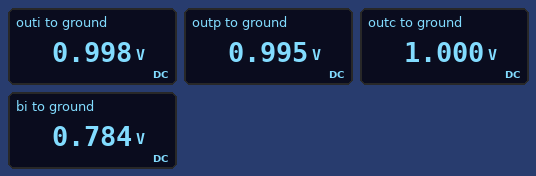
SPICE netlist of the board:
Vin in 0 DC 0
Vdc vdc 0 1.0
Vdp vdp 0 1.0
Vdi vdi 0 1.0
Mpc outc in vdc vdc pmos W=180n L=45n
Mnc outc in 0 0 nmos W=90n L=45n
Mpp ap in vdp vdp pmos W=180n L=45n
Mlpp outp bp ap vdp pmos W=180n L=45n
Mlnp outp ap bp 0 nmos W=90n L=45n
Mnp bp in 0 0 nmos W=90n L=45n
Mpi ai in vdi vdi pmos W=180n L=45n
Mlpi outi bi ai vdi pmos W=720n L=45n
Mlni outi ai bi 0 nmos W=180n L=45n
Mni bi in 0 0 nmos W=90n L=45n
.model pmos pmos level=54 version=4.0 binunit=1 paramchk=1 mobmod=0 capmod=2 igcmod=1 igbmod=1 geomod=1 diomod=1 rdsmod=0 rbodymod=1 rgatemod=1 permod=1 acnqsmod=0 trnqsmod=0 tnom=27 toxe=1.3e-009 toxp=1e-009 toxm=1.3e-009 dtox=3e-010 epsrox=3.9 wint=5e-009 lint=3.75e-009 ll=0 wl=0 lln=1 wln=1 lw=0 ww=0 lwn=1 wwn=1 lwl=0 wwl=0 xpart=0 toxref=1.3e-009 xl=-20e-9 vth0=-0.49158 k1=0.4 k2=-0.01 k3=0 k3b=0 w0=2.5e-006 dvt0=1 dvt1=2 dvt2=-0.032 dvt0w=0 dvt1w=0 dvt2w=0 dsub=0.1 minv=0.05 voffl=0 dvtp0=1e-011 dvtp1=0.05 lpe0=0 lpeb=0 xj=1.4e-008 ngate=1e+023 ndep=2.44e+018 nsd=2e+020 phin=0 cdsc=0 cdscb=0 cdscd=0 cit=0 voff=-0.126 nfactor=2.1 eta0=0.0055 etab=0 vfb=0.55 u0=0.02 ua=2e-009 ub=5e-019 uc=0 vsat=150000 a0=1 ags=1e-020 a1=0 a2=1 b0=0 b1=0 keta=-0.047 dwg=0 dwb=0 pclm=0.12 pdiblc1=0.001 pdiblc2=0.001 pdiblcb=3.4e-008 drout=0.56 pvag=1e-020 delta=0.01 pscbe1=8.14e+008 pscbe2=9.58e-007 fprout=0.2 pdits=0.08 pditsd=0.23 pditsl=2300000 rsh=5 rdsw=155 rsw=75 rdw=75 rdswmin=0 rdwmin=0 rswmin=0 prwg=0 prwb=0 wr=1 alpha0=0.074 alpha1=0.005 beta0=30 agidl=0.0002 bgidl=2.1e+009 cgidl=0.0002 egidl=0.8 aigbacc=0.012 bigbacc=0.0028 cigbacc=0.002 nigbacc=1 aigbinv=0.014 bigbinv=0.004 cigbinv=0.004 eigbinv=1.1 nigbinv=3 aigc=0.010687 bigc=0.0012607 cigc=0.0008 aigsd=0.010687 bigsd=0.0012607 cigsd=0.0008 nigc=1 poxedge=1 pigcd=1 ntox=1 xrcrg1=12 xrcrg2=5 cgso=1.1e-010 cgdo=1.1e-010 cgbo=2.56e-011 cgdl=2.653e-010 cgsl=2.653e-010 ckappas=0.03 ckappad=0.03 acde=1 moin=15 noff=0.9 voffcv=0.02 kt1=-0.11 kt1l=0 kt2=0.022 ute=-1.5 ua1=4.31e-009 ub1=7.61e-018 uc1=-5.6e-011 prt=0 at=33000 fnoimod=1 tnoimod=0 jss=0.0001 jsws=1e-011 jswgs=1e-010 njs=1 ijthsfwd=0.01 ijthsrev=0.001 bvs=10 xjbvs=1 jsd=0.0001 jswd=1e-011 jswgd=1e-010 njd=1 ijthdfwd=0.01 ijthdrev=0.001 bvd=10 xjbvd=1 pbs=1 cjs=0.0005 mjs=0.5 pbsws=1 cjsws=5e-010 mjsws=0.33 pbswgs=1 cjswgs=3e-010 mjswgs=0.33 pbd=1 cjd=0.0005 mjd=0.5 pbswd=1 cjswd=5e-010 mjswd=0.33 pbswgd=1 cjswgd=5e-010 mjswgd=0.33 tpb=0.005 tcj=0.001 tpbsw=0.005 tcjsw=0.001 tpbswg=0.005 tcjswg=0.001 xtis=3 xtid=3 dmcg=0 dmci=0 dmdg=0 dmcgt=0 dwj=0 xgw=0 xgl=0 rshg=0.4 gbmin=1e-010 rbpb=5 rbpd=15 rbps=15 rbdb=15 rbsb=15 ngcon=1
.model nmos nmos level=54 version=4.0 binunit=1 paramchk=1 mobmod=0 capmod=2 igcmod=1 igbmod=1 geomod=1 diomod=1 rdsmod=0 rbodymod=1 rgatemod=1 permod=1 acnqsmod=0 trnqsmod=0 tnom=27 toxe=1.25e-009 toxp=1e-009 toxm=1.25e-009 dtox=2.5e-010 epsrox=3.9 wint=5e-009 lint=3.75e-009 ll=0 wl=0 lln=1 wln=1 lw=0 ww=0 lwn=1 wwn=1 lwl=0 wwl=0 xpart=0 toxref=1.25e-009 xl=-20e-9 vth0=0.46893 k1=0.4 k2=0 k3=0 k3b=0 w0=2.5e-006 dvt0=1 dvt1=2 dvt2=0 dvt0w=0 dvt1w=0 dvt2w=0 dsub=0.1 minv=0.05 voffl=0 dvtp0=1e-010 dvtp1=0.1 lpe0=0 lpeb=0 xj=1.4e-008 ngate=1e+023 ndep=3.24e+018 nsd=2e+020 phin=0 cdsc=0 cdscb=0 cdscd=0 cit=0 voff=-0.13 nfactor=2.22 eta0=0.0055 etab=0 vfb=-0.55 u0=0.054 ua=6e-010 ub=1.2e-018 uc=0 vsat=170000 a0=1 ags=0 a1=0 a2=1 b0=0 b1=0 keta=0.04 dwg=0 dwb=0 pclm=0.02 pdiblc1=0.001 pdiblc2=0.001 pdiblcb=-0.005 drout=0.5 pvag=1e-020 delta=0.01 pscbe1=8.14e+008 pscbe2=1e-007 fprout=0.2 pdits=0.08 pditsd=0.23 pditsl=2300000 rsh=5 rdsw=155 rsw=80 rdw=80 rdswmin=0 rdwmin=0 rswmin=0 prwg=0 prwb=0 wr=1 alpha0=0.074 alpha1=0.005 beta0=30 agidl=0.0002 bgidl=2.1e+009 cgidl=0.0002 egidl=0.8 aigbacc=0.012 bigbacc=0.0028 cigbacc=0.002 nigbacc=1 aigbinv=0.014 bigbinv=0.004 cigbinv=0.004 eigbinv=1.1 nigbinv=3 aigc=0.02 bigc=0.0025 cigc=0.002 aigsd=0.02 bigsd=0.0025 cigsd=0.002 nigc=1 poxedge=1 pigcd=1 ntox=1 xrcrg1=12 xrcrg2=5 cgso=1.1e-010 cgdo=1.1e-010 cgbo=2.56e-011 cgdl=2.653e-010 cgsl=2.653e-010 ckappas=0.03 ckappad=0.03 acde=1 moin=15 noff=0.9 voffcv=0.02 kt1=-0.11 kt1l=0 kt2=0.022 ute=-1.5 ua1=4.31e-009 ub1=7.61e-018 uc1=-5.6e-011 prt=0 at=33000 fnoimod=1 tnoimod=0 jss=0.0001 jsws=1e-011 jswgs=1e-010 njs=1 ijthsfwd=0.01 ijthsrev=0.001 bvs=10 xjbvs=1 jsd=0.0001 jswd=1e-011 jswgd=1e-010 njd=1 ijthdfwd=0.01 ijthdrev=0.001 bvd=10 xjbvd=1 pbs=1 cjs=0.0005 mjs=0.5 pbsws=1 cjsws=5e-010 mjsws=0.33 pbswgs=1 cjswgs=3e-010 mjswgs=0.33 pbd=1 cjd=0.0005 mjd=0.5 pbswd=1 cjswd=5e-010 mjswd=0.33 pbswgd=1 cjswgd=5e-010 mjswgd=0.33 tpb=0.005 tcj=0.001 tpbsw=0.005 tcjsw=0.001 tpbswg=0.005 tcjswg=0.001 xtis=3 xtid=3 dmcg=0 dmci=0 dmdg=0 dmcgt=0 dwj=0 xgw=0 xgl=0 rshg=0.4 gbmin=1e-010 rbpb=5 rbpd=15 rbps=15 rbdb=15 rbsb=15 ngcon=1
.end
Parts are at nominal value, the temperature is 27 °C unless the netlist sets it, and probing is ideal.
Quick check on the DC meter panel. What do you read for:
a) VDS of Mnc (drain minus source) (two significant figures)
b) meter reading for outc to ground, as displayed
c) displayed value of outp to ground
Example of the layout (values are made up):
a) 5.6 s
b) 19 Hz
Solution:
a) 1.0 V
b) 1.000 V
c) 0.995 V
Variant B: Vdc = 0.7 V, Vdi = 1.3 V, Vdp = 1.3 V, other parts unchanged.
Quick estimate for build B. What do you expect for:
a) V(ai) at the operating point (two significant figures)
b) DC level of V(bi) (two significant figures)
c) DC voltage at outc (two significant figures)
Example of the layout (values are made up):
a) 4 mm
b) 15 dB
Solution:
a) 1.3 V
b) 1.0 V
c) 700 mV
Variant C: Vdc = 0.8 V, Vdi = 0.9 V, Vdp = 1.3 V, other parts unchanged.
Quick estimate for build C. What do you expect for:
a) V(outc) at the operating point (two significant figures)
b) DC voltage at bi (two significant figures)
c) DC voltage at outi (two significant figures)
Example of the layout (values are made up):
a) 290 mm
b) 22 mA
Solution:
a) 800 mV
b) 700 mV
c) 900 mV
